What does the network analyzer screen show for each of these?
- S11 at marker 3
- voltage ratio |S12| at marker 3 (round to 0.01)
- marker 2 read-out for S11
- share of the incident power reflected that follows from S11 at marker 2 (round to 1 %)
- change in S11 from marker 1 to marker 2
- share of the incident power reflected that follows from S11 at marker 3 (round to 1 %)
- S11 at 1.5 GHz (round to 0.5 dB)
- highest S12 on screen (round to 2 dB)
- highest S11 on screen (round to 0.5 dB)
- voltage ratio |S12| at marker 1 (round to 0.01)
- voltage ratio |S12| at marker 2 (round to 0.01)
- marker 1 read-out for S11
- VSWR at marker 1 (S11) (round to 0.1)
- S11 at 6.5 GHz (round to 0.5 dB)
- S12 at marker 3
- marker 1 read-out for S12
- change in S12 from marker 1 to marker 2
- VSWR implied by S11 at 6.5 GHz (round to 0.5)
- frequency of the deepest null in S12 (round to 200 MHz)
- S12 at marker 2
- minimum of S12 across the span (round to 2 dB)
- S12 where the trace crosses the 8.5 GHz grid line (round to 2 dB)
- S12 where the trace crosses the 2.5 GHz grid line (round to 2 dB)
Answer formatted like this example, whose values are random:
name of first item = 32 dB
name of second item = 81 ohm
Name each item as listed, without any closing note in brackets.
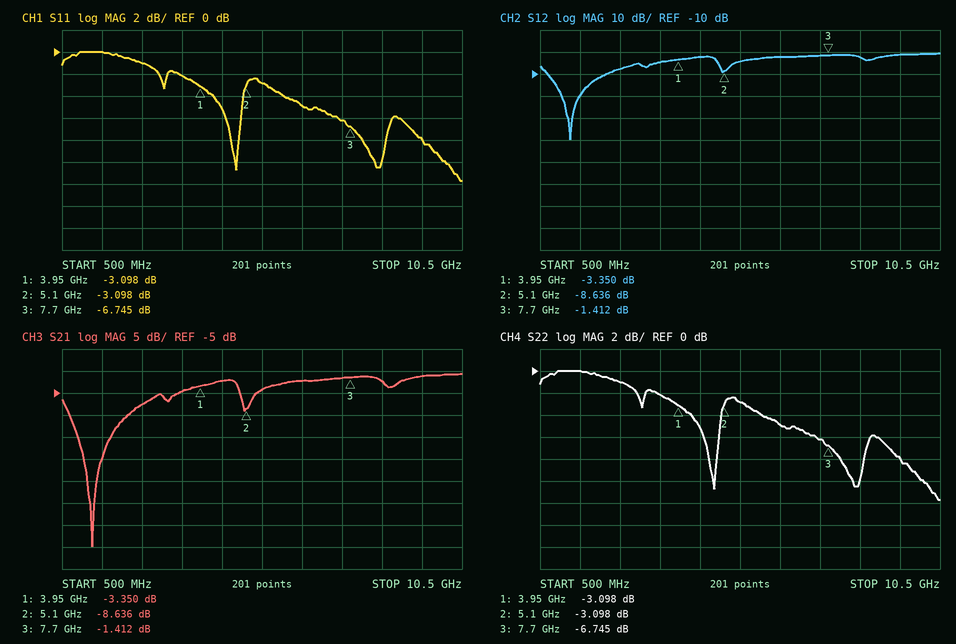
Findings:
S11 at marker 3 = -6.745 dB
voltage ratio |S12| at marker 3 = 0.85
marker 2 read-out for S11 = -3.098 dB
share of the incident power reflected that follows from S11 at marker 2 = 49 %
change in S11 from marker 1 to marker 2 = 0.000 dB
share of the incident power reflected that follows from S11 at marker 3 = 21 %
S11 at 1.5 GHz = 0.0 dB
highest S12 on screen = 0 dB
highest S11 on screen = 0.0 dB
voltage ratio |S12| at marker 1 = 0.68
voltage ratio |S12| at marker 2 = 0.37
marker 1 read-out for S11 = -3.098 dB
VSWR at marker 1 (S11) = 5.7
S11 at 6.5 GHz = -5.0 dB
S12 at marker 3 = -1.412 dB
marker 1 read-out for S12 = -3.350 dB
change in S12 from marker 1 to marker 2 = -5.286 dB
VSWR implied by S11 at 6.5 GHz = 3.5
frequency of the deepest null in S12 = 1.2 GHz
S12 at marker 2 = -8.636 dB
minimum of S12 across the span = -40 dB
S12 where the trace crosses the 8.5 GHz grid line = -2 dB
S12 where the trace crosses the 2.5 GHz grid line = -8 dB
